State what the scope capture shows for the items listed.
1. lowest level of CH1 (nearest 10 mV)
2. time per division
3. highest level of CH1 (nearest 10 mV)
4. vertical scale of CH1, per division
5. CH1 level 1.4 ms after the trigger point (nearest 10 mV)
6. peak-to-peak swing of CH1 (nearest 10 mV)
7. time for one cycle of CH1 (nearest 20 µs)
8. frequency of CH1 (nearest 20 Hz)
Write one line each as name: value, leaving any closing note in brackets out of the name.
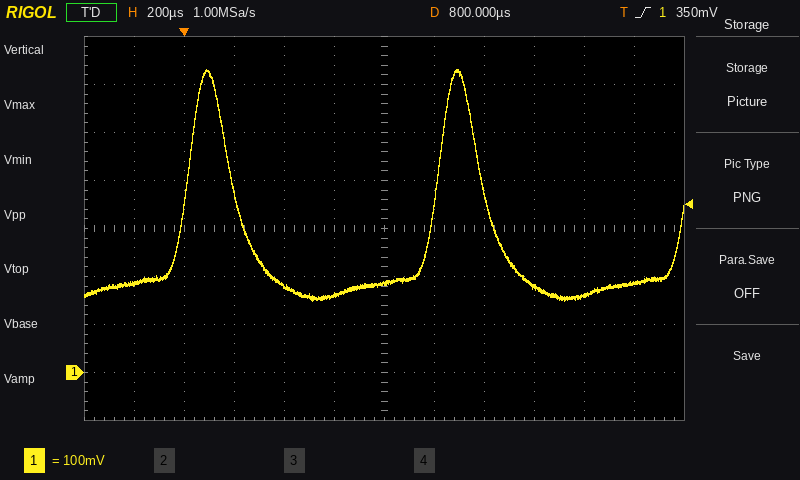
lowest level of CH1: 150 mV
time per division: 200 µs
highest level of CH1: 630 mV
vertical scale of CH1, per division: 100 mV
CH1 level 1.4 ms after the trigger point: 180 mV
peak-to-peak swing of CH1: 480 mV
time for one cycle of CH1: 1.00 ms
frequency of CH1: 1.00 kHz
